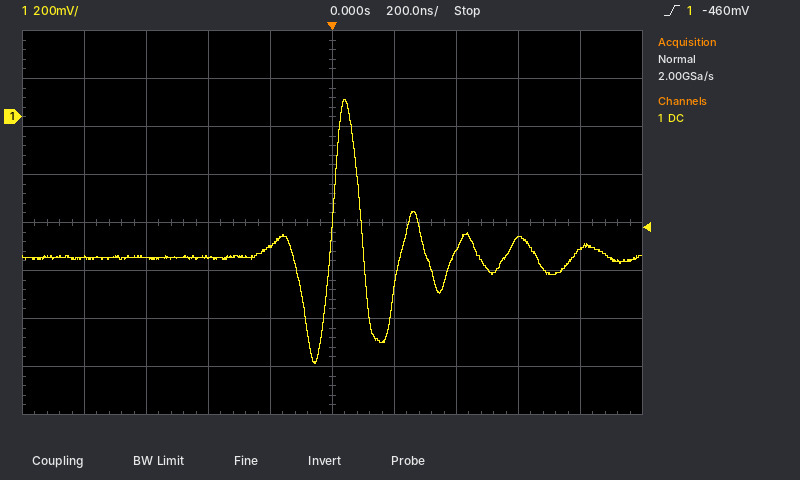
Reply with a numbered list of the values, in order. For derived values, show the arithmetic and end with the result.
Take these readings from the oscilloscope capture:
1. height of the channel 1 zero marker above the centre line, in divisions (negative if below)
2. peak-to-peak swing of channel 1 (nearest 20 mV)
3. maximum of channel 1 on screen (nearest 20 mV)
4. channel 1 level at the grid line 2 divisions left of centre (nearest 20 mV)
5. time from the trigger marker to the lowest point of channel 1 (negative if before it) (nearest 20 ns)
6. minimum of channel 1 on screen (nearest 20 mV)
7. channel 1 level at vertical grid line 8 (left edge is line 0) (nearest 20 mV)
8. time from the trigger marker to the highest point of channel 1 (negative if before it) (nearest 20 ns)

1. +2.2 div
2. 80 mV − (-1.02 V) = 1.10 V
3. 80 mV
4. -580 mV
5. -60 ns
6. -1.02 V
7. -500 mV
8. +40 ns
